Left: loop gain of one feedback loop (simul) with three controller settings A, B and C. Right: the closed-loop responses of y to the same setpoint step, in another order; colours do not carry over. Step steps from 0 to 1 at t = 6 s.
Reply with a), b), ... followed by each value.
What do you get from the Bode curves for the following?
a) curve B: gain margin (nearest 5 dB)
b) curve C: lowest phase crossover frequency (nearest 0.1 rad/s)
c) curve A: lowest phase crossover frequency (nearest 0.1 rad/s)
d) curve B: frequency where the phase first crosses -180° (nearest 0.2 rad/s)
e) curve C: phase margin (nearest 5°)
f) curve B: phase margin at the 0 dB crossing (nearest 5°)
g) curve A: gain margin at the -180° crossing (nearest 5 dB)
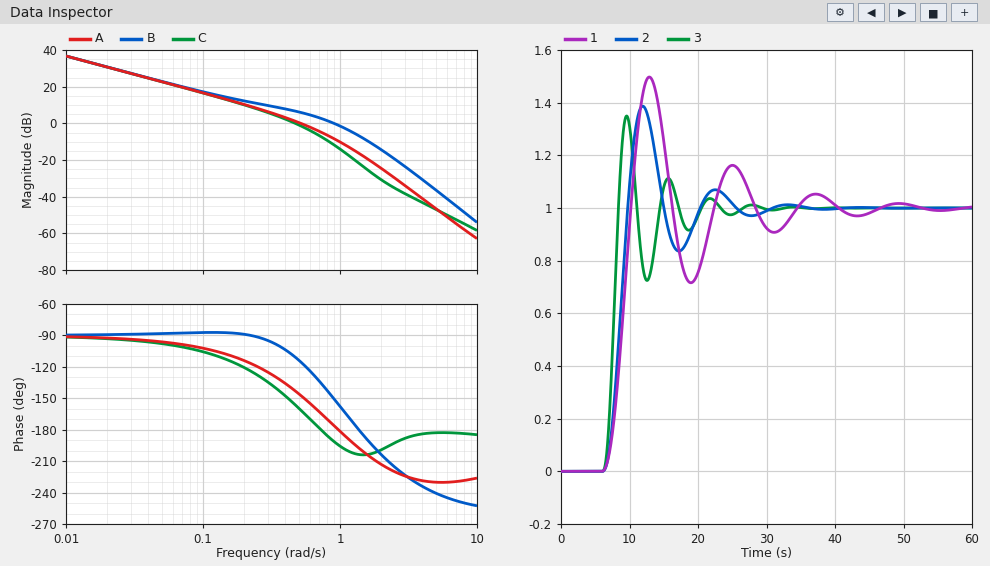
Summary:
a) 5 dB
b) 0.7 rad/s
c) 1.0 rad/s
d) 1.4 rad/s
e) 25°
f) 30°
g) 10 dB
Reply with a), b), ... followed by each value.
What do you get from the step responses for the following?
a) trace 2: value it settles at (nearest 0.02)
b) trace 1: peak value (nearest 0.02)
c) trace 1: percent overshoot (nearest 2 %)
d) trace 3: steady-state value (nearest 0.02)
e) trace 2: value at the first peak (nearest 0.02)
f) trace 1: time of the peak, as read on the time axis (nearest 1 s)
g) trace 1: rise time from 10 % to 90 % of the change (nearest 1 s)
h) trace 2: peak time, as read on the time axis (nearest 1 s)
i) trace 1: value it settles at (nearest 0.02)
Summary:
a) 1.00
b) 1.50
c) 50 %
d) 1.00
e) 1.38
f) 13 s
g) 3 s
h) 12 s
i) 1.00
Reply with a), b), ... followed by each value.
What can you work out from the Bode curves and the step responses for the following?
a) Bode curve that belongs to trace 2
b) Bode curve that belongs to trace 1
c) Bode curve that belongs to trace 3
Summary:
a) A
b) C
c) B
